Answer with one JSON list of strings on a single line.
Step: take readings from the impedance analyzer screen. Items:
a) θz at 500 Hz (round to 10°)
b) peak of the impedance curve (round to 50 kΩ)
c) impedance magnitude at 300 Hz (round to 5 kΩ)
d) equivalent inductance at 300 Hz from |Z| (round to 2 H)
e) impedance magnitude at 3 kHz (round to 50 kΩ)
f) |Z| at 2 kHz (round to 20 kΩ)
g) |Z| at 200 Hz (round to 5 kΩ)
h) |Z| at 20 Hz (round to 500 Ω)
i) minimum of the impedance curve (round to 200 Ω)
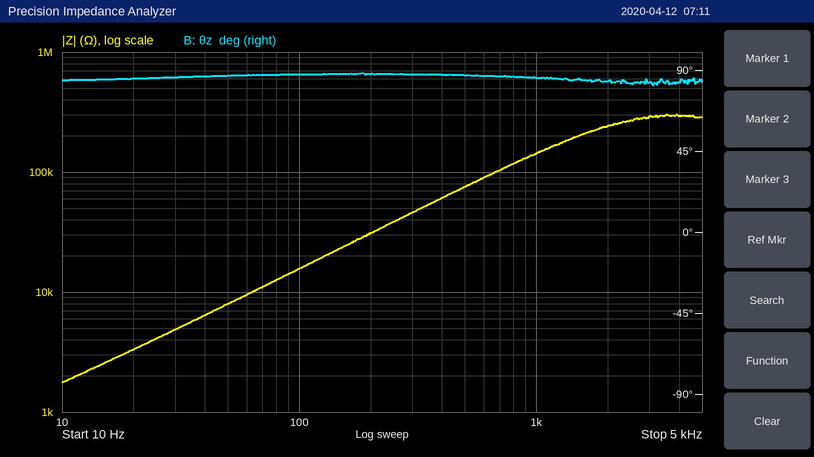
["90°", "300 kΩ", "45 kΩ", "24 H", "300 kΩ", "240 kΩ", "30 kΩ", "3.5 kΩ", "1.8 kΩ"]
